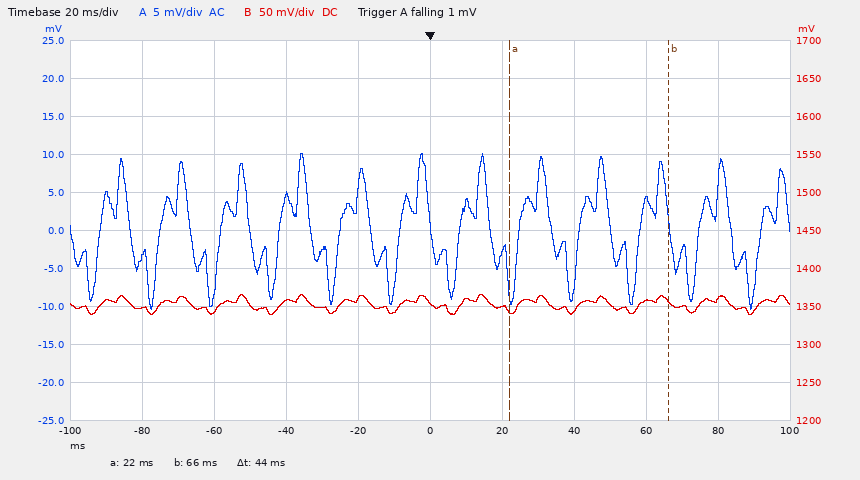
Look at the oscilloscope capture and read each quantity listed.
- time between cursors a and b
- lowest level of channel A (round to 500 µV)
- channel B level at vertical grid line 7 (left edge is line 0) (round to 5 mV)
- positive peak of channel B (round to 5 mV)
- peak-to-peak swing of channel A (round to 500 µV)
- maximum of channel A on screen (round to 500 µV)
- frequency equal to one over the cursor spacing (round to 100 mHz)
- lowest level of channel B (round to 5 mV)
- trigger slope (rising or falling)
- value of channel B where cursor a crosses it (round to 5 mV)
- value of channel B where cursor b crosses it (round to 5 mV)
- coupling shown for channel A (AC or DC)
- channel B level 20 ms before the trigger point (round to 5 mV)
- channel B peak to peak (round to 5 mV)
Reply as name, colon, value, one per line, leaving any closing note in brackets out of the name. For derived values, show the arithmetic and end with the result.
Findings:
time between cursors a and b: 44 ms
lowest level of channel A: -10.5 mV
channel B level at vertical grid line 7 (left edge is line 0): 1.345 V
positive peak of channel B: 1.365 V
peak-to-peak swing of channel A: 10.0 mV − (-10.5 mV) = 20.5 mV
maximum of channel A on screen: 10.0 mV
frequency equal to one over the cursor spacing: 1 / 44 ms ≈ 22.7 Hz
lowest level of channel B: 1.340 V
trigger slope: falling
value of channel B where cursor a crosses it: 1.345 V
value of channel B where cursor b crosses it: 1.355 V
coupling shown for channel A: AC
channel B level 20 ms before the trigger point: 1.360 V
channel B peak to peak: 1.365 V − (1.340 V) = 25 mV
